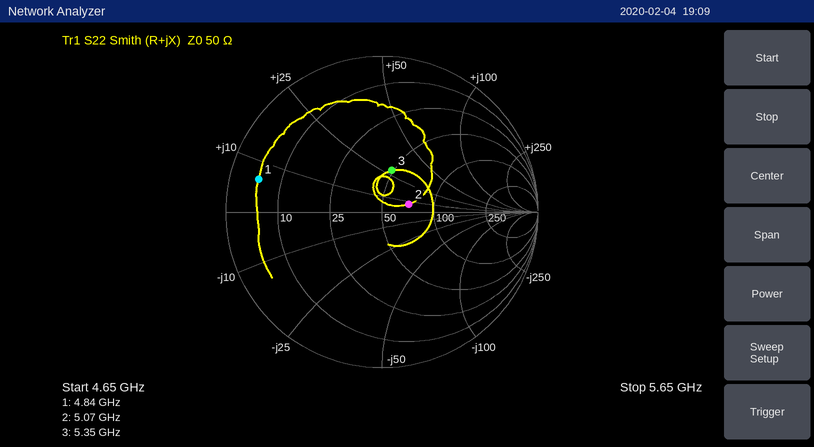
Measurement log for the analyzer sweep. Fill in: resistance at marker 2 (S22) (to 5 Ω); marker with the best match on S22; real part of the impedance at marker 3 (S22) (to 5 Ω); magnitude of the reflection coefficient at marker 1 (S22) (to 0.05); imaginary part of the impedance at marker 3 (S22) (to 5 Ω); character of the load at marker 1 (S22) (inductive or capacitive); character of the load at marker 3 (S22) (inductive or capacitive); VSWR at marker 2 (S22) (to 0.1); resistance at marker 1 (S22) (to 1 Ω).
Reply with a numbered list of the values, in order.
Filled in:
1. 70 Ω
2. marker 2
3. 50 Ω
4. 0.80
5. +30 Ω
6. inductive
7. inductive
8. 1.4
9. 5 Ω
